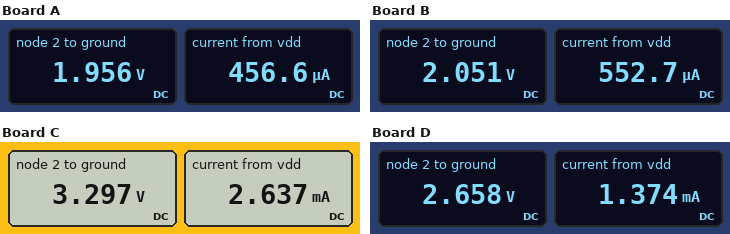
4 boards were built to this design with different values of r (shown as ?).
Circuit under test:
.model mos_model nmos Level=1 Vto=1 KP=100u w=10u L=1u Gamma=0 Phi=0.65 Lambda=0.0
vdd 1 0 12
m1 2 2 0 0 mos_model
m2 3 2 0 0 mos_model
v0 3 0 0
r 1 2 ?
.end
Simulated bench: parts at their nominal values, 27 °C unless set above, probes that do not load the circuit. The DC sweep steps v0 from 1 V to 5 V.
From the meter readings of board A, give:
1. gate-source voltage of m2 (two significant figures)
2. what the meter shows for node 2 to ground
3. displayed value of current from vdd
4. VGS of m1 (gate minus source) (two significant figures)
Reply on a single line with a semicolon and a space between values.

2.0 V; 1.956 V; 456.6 µA; 2.0 V
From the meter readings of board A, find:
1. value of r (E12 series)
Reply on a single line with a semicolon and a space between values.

22 kΩ
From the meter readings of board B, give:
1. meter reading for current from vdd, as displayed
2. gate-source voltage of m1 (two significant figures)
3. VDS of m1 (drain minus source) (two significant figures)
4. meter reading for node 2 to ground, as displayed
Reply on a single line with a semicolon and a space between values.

552.7 µA; 2.1 V; 2.1 V; 2.051 V
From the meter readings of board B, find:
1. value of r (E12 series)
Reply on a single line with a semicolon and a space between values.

18 kΩ
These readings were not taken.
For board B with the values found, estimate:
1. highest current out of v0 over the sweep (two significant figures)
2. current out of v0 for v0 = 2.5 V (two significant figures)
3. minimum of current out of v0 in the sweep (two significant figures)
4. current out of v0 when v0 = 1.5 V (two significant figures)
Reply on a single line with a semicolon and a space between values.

550 µA; 550 µA; 550 µA; 550 µA
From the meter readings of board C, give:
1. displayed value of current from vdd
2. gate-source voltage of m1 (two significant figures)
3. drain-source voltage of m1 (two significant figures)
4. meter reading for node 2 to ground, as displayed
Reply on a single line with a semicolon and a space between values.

2.637 mA; 3.3 V; 3.3 V; 3.297 V
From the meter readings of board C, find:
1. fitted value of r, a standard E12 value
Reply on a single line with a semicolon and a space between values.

3.3 kΩ
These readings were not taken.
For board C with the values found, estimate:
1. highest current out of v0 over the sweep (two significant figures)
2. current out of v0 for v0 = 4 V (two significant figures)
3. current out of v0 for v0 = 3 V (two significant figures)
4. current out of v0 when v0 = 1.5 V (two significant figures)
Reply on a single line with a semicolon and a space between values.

2.6 mA; 2.6 mA; 2.6 mA; 2.3 mA
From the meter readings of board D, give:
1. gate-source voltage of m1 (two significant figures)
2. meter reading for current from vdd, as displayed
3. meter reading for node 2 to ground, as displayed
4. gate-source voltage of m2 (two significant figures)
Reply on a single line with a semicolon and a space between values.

2.7 V; 1.374 mA; 2.658 V; 2.7 V
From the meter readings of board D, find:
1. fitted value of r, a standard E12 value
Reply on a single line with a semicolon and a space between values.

6.8 kΩ
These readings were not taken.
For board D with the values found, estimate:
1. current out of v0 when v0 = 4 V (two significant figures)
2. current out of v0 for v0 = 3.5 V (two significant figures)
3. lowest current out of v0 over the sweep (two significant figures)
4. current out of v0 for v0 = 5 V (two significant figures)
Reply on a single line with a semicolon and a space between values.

1.4 mA; 1.4 mA; 1.2 mA; 1.4 mA
